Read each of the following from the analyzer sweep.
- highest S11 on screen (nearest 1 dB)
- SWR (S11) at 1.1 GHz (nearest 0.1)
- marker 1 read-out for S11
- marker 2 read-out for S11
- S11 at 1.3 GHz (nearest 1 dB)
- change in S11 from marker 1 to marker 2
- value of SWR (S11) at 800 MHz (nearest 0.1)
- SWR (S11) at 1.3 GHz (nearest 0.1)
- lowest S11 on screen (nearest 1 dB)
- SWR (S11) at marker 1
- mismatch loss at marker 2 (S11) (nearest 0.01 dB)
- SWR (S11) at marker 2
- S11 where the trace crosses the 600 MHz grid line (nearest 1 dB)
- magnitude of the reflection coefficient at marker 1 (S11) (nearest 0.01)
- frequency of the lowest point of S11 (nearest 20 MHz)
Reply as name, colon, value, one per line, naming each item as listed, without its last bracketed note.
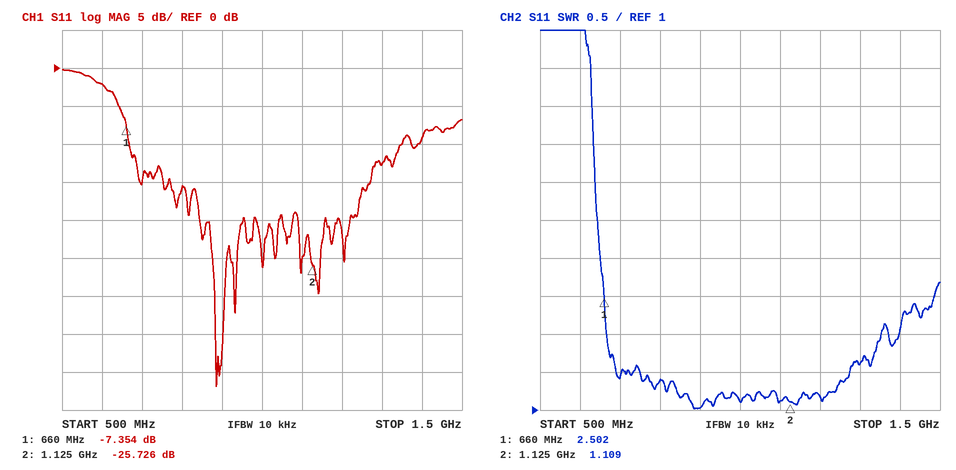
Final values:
highest S11 on screen: 0 dB
SWR (S11) at 1.1 GHz: 1.1
marker 1 read-out for S11: -7.354 dB
marker 2 read-out for S11: -25.726 dB
S11 at 1.3 GHz: -13 dB
change in S11 from marker 1 to marker 2: -18.372 dB
value of SWR (S11) at 800 MHz: 1.4
SWR (S11) at 1.3 GHz: 1.6
lowest S11 on screen: -42 dB
SWR (S11) at marker 1: 2.502
mismatch loss at marker 2 (S11): 0.01 dB
SWR (S11) at marker 2: 1.109
S11 where the trace crosses the 600 MHz grid line: -2 dB
magnitude of the reflection coefficient at marker 1 (S11): 0.43
frequency of the lowest point of S11: 880 MHz
